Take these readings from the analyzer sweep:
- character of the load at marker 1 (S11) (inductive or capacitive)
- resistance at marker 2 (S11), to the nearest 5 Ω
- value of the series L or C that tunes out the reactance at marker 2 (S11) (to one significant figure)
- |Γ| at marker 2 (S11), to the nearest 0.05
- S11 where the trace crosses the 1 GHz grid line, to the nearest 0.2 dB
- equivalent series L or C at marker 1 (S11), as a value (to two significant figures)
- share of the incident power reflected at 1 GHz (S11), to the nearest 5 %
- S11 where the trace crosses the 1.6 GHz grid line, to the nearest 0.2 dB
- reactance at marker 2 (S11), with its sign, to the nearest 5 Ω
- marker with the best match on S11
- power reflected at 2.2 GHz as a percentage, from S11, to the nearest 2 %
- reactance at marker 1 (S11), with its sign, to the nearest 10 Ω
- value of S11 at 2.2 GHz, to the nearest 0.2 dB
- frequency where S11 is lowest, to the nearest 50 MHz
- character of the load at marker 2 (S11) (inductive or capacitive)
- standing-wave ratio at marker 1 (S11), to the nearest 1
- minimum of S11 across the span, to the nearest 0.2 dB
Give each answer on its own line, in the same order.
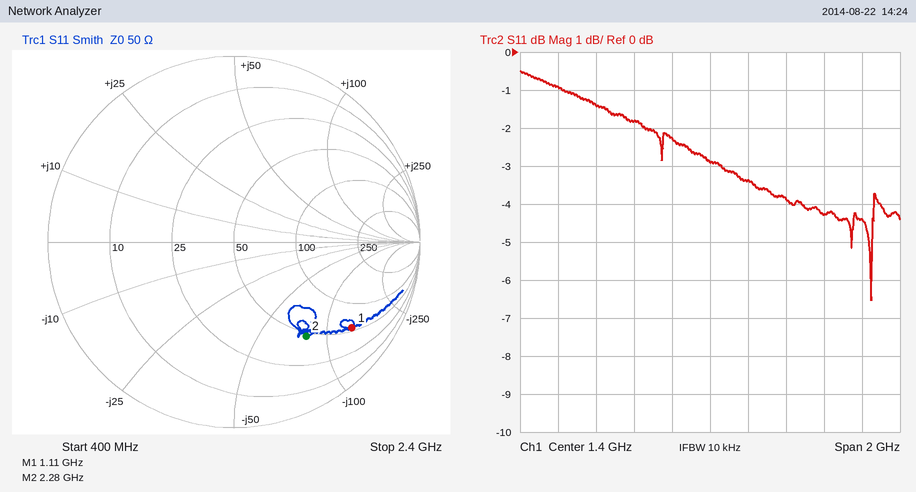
capacitive
45 Ω
6 nH
0.65
-1.8 dB
1.1 pF
65 %
-3.4 dB
-80 Ω
marker 2
36 %
-130 Ω
-4.4 dB
2.25 GHz
capacitive
8
-6.6 dB
